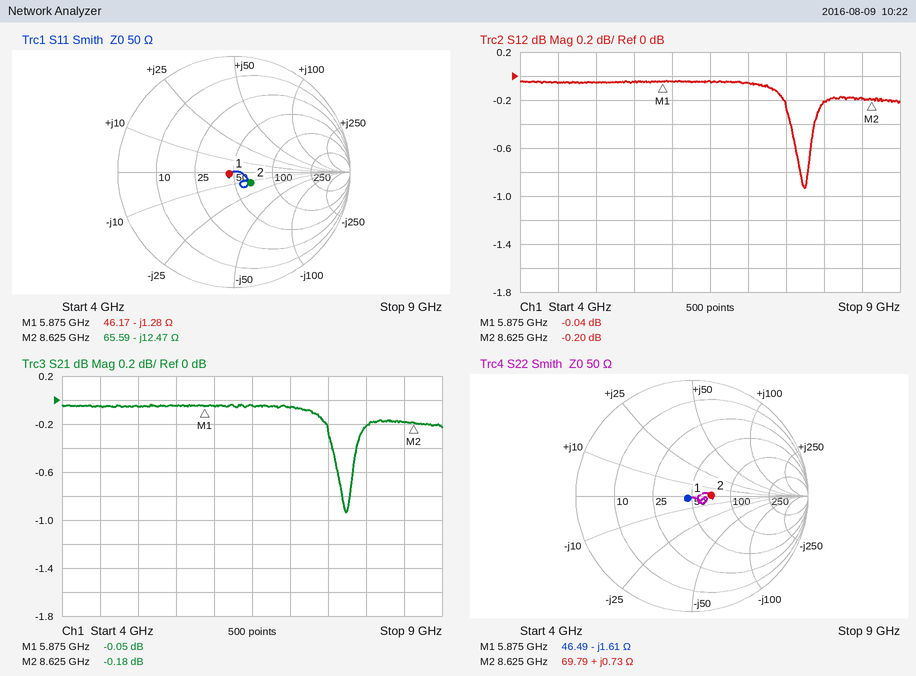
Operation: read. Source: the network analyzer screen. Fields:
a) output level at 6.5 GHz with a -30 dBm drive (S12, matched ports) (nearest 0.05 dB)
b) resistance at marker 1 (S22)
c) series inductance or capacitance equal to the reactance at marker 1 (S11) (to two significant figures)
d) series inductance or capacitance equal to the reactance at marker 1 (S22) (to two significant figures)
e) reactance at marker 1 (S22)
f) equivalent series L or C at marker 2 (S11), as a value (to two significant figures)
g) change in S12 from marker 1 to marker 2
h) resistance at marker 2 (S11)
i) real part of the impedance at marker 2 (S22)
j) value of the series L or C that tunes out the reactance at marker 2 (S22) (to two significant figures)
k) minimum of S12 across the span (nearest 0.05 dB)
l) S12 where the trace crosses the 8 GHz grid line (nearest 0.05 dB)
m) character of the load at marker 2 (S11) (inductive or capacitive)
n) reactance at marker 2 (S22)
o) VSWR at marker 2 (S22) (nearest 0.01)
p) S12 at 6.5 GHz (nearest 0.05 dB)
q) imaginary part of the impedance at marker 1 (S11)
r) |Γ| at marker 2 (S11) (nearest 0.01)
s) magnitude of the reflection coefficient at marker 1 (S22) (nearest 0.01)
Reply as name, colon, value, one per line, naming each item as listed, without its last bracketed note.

output level at 6.5 GHz with a -30 dBm drive (S12, matched ports): -30.05 dBm
resistance at marker 1: 46.49 Ω
series inductance or capacitance equal to the reactance at marker 1 (S11): 21 pF
series inductance or capacitance equal to the reactance at marker 1 (S22): 17 pF
reactance at marker 1: -1.61 Ω
equivalent series L or C at marker 2 (S11), as a value: 1.5 pF
change in S12 from marker 1 to marker 2: -0.16 dB
resistance at marker 2: 65.59 Ω
real part of the impedance at marker 2: 69.79 Ω
value of the series L or C that tunes out the reactance at marker 2 (S22): 25 pF
minimum of S12 across the span: -0.95 dB
S12 where the trace crosses the 8 GHz grid line: -0.20 dB
character of the load at marker 2 (S11): capacitive
reactance at marker 2: +0.73 Ω
VSWR at marker 2 (S22): 1.40
S12 at 6.5 GHz: -0.05 dB
imaginary part of the impedance at marker 1: -1.28 Ω
|Γ| at marker 2 (S11): 0.17
magnitude of the reflection coefficient at marker 1 (S22): 0.04
